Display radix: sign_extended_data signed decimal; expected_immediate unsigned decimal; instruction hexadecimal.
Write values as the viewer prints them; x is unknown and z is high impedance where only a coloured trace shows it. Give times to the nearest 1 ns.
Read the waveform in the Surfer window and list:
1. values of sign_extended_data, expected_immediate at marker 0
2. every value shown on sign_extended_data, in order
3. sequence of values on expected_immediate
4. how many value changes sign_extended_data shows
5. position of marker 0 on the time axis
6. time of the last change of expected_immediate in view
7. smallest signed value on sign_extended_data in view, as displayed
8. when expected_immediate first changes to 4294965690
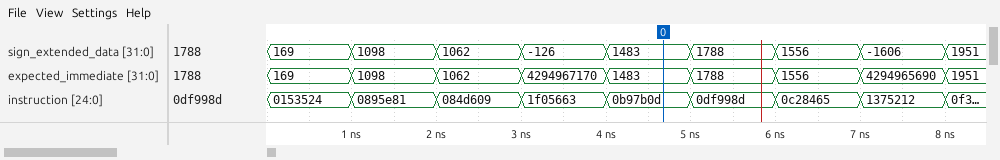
sign_extended_data=1483, expected_immediate=1483
169, 1098, 1062, -126, 1483, 1788, 1556, -1606, 1951
169, 1098, 1062, 4294967170, 1483, 1788, 1556, 4294965690, 1951
8
5 ns
8 ns
-1606
7 ns
